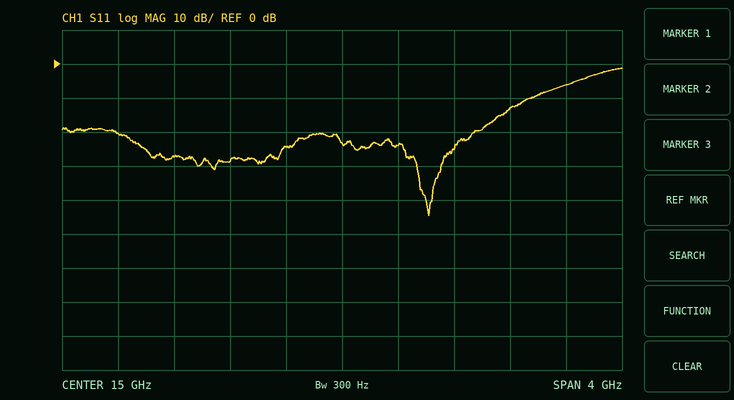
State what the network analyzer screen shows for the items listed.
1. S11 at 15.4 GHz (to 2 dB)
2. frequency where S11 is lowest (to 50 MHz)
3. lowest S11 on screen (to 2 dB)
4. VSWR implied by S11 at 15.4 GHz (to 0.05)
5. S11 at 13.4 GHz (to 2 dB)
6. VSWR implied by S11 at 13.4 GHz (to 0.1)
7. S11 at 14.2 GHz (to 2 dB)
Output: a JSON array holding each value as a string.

["-24 dB", "15.60 GHz", "-44 dB", "1.15", "-20 dB", "1.2", "-28 dB"]
